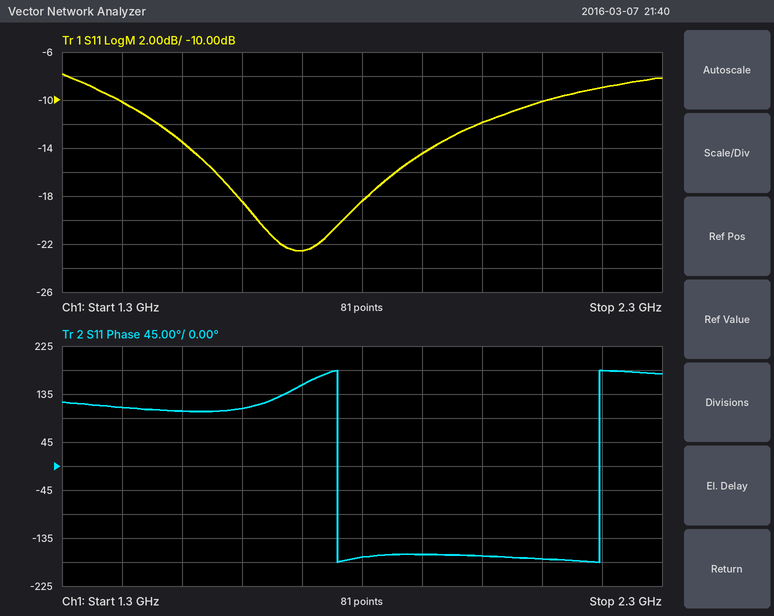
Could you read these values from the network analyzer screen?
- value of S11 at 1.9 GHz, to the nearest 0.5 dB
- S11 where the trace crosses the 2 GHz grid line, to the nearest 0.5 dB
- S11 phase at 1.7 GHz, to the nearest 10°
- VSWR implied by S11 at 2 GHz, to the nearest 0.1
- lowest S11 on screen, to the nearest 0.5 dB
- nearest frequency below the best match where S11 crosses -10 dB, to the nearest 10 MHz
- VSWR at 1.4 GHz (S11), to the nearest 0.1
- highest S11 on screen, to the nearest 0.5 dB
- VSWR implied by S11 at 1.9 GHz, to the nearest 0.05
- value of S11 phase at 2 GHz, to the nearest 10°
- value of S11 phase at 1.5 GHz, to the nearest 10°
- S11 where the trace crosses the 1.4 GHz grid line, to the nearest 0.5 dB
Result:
-14.5 dB
-12.0 dB
150°
1.7
-22.5 dB
1.39 GHz
1.9
-8.0 dB
1.45
-170°
100°
-10.0 dB
